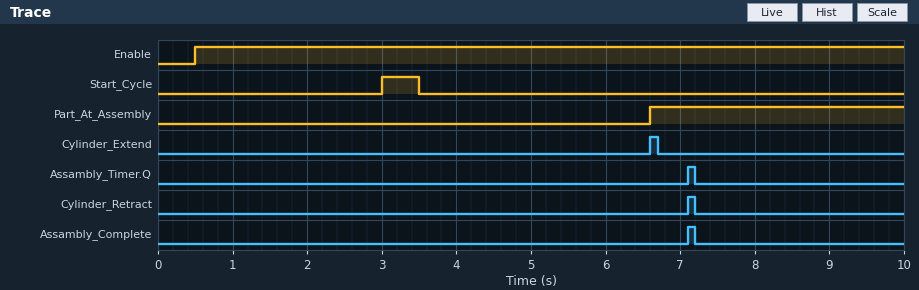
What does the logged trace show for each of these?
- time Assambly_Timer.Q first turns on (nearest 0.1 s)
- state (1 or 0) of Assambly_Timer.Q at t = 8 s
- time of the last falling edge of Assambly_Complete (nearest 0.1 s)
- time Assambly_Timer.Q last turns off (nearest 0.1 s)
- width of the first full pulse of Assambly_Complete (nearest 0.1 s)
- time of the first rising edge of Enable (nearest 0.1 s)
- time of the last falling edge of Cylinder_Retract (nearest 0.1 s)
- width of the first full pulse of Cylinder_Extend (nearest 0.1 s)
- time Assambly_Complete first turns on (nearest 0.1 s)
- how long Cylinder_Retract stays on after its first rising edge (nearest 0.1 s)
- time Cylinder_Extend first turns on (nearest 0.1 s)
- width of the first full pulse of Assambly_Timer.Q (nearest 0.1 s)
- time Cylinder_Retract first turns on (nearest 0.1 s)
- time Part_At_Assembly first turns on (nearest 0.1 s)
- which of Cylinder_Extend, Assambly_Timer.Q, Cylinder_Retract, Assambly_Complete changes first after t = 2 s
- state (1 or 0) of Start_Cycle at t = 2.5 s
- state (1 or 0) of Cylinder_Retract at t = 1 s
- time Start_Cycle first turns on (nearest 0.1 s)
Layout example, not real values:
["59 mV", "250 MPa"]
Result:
["7.1 s", "0", "7.2 s", "7.2 s", "0.1 s", "0.5 s", "7.2 s", "0.1 s", "7.1 s", "0.1 s", "6.6 s", "0.1 s", "7.1 s", "6.6 s", "Cylinder_Extend", "0", "0", "3.0 s"]
